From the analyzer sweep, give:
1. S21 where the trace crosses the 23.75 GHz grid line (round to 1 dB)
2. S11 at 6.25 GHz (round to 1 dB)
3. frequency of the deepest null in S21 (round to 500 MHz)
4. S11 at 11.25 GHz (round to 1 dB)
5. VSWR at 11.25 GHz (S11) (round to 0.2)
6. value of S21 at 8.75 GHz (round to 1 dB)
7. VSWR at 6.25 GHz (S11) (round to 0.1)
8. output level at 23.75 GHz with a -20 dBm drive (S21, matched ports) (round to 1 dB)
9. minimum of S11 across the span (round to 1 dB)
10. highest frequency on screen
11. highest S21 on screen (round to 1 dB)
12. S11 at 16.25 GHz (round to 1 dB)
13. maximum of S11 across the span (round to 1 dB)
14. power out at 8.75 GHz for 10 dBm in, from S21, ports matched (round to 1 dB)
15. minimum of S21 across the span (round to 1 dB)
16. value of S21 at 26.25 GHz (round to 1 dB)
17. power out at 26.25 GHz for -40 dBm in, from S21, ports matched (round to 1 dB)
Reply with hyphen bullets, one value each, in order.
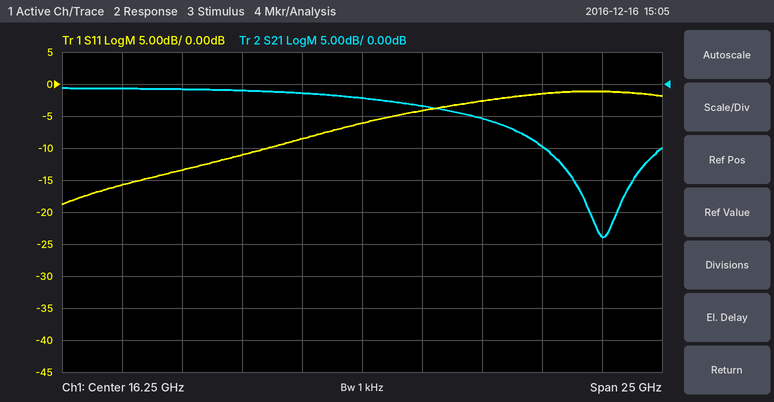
- -10 dB
- -16 dB
- 26.5 GHz
- -11 dB
- 1.8
- -1 dB
- 1.4
- -30 dBm
- -19 dB
- 28.75 GHz
- -1 dB
- -6 dB
- -1 dB
- 9 dBm
- -24 dB
- -24 dB
- -64 dBm
